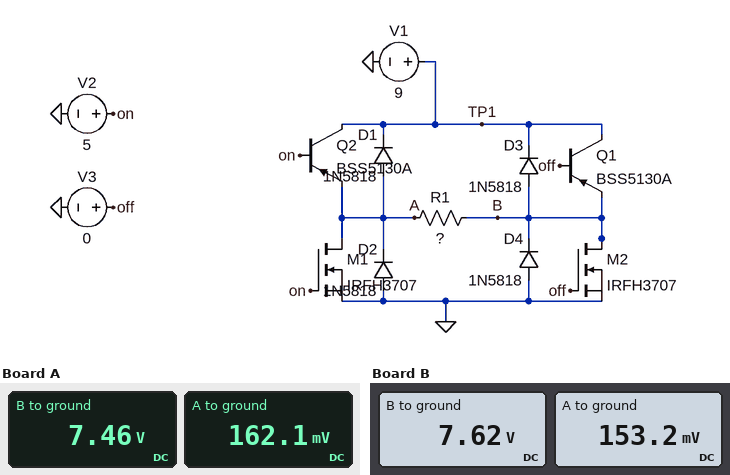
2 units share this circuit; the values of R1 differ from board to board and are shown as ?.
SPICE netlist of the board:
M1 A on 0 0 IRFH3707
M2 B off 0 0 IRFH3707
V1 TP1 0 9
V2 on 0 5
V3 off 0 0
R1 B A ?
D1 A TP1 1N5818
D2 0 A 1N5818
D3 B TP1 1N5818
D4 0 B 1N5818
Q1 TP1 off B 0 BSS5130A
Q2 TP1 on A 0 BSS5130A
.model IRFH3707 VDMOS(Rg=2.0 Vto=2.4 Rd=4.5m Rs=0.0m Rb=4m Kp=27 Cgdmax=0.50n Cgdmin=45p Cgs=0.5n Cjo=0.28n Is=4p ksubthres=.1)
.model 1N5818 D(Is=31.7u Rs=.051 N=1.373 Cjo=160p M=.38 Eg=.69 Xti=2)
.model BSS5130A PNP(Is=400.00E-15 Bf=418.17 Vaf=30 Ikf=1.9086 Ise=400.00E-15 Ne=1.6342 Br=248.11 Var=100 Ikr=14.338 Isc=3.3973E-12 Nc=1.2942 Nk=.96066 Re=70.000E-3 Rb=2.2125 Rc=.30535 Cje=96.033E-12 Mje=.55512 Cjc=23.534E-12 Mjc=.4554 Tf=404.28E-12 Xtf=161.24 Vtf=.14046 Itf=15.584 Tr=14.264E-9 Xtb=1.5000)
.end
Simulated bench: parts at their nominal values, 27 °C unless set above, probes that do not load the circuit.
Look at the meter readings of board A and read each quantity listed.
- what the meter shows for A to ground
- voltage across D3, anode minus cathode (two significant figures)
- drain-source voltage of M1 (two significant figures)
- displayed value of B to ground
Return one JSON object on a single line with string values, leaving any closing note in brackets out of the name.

{"what the meter shows for A to ground": "162.1 mV", "voltage across D3, anode minus cathode": "-1.5 V", "drain-source voltage of M1": "160 mV", "displayed value of B to ground": "7.46 V"}
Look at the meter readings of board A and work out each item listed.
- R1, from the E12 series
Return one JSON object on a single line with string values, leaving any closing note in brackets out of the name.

{"R1, from the E12 series": "4.7 Ω"}
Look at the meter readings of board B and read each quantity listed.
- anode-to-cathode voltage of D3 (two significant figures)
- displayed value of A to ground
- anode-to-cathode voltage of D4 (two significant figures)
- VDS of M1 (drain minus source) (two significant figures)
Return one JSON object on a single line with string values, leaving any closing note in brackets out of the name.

{"anode-to-cathode voltage of D3": "-1.4 V", "displayed value of A to ground": "153.2 mV", "anode-to-cathode voltage of D4": "-7.6 V", "VDS of M1 (drain minus source)": "150 mV"}
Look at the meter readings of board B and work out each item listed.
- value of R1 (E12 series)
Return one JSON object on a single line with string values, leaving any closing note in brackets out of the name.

{"value of R1": "6.8 Ω"}
